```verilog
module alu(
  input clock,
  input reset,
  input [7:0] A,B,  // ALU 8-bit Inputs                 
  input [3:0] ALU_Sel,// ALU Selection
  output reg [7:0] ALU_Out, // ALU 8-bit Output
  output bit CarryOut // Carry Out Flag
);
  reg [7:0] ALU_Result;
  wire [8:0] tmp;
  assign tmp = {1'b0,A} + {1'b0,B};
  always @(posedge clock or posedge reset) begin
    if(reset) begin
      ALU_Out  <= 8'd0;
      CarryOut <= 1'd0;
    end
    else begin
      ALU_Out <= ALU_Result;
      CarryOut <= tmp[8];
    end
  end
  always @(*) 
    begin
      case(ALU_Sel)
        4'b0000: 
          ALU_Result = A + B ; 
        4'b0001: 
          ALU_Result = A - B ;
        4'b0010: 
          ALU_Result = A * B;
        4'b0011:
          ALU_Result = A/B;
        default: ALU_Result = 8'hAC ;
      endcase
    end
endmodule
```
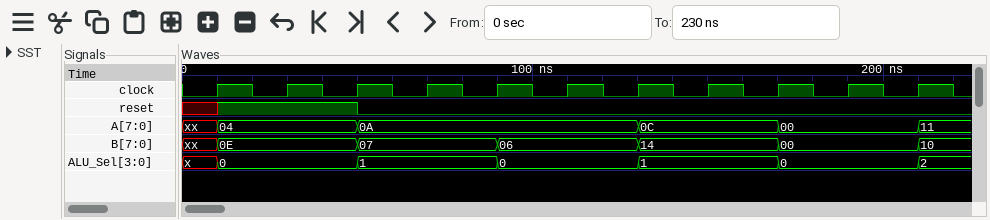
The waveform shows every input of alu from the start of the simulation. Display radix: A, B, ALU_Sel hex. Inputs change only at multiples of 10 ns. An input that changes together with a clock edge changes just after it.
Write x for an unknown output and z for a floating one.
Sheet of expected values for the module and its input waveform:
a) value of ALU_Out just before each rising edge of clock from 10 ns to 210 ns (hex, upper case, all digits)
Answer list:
x, 00, 00, 00, 03, 03, 10, 10, F8, F8, 00
